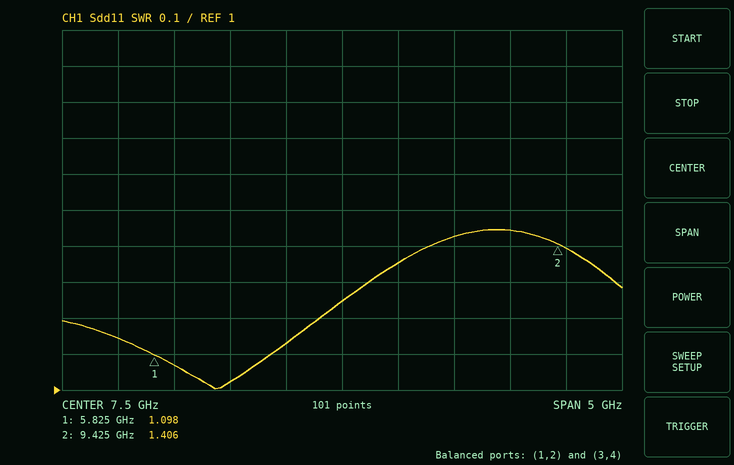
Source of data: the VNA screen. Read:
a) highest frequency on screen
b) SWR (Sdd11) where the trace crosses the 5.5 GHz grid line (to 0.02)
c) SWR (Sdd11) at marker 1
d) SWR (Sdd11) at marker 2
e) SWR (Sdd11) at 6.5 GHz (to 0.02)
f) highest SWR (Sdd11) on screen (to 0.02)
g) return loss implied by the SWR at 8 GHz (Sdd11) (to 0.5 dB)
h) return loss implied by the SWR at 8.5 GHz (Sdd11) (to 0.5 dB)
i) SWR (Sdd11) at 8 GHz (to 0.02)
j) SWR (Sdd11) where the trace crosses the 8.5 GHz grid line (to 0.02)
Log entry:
10 GHz
1.14
1.098
1.406
1.02
1.44
16.5 dB
15.0 dB
1.36
1.42
